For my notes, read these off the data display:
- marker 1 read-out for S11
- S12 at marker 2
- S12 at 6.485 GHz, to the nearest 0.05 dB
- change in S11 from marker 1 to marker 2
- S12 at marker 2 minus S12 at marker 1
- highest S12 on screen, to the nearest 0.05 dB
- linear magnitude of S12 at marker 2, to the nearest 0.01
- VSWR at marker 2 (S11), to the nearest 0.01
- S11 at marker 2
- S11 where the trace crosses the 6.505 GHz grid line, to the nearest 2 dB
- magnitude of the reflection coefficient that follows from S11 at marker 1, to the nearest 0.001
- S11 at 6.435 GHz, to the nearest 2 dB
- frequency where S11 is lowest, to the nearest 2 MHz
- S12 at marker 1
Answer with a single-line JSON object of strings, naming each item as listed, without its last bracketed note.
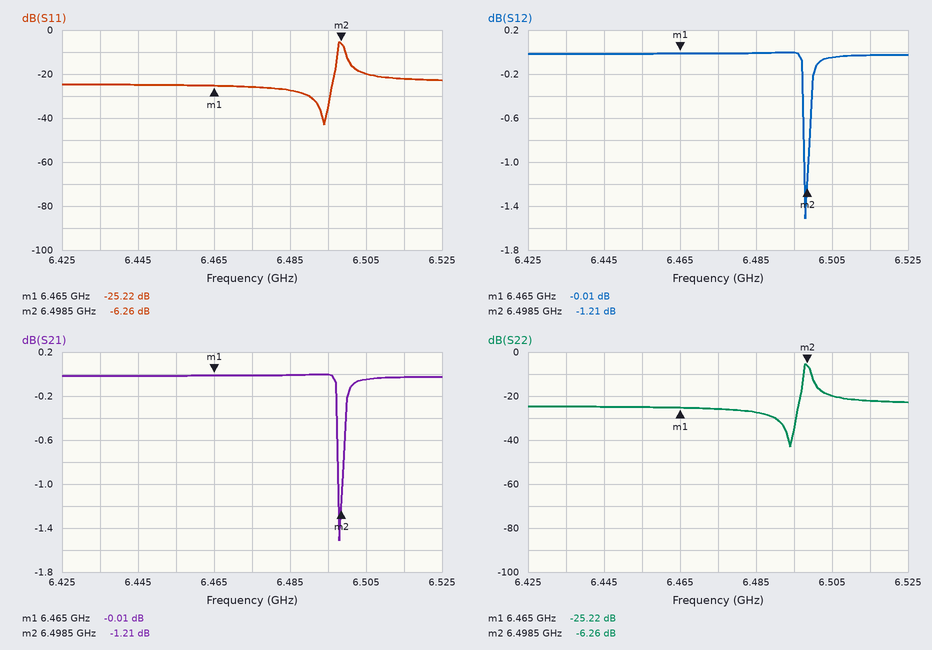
{"marker 1 read-out for S11": "-25.22 dB", "S12 at marker 2": "-1.21 dB", "S12 at 6.485 GHz, to the nearest 0.05 dB": "0.00 dB", "change in S11 from marker 1 to marker 2": "18.96 dB", "S12 at marker 2 minus S12 at marker 1": "-1.20 dB", "highest S12 on screen, to the nearest 0.05 dB": "0.00 dB", "linear magnitude of S12 at marker 2, to the nearest 0.01": "0.87", "VSWR at marker 2 (S11), to the nearest 0.01": "2.89", "S11 at marker 2": "-6.26 dB", "S11 where the trace crosses the 6.505 GHz grid line, to the nearest 2 dB": "-20 dB", "magnitude of the reflection coefficient that follows from S11 at marker 1, to the nearest 0.001": "0.055", "S11 at 6.435 GHz, to the nearest 2 dB": "-24 dB", "frequency where S11 is lowest, to the nearest 2 MHz": "6.494 GHz", "S12 at marker 1": "-0.01 dB"}
